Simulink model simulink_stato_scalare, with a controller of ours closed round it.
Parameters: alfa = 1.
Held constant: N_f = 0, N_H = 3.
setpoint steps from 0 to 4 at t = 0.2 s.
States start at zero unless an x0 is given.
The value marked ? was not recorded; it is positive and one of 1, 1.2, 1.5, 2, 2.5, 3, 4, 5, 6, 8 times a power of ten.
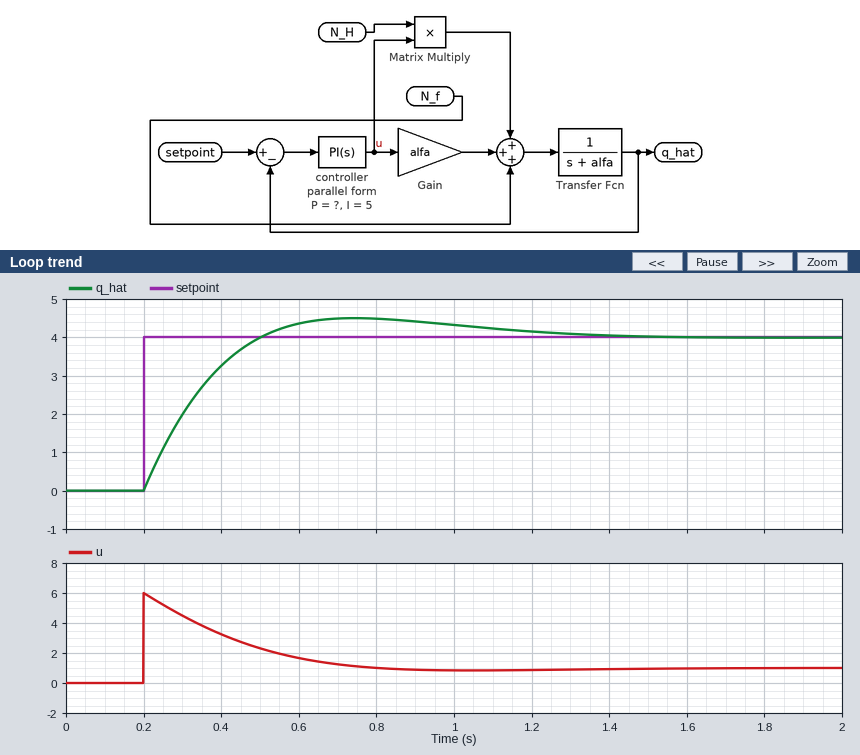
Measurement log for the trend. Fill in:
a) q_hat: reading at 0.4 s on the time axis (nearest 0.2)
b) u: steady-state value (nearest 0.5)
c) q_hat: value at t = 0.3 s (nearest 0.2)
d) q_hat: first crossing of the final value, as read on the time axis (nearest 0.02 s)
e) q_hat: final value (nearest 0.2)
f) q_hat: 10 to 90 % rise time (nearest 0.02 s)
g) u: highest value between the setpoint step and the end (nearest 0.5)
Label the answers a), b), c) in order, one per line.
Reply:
a) 3.2
b) 1.0
c) 2.0
d) 0.50 s
e) 4.0
f) 0.22 s
g) 6.0
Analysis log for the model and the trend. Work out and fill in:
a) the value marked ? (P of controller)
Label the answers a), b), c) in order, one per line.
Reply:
a) 1.5
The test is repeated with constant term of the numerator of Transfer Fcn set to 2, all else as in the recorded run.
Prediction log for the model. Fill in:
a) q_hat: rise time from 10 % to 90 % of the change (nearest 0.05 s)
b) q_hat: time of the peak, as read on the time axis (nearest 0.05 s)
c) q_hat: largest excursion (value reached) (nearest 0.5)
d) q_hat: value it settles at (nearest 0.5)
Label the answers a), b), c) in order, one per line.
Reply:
a) 0.15 s
b) 0.55 s
c) 4.5
d) 4.0
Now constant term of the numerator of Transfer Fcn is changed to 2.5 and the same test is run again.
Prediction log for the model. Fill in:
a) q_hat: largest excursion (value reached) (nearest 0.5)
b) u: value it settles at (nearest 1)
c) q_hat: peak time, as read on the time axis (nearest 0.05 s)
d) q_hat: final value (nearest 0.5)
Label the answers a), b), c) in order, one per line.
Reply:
a) 4.5
b) 0
c) 0.50 s
d) 4.0
